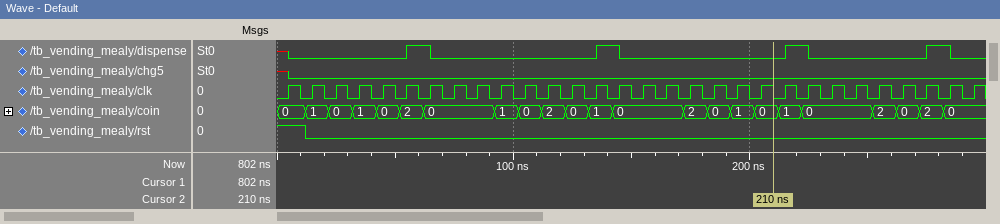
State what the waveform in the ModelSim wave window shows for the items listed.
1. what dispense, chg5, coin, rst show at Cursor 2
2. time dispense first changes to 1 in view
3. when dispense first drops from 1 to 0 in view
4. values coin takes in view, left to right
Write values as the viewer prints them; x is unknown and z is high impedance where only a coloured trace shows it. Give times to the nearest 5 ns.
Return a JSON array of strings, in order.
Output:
["dispense=0, chg5=0, coin=0, rst=0", "55 ns", "65 ns", "0, 1, 0, 1, 0, 2, 0, 1, 0, 2, 0, 1, 0, 2, 0, 1, 0, 1, 0, 2, 0, 2, 0"]
